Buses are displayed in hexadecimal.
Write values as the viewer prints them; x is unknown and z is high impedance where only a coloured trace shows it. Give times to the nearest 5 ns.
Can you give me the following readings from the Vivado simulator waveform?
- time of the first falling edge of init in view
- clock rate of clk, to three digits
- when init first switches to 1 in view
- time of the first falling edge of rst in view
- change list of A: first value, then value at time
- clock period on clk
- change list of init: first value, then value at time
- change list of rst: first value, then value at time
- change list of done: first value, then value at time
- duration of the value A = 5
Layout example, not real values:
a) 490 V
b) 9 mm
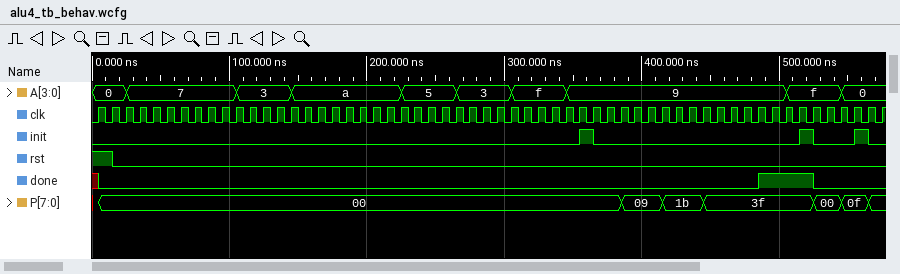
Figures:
a) 365 ns
b) 100 MHz
c) 355 ns
d) 15 ns
e) 0, 7 at 25 ns, 3 at 105 ns, a at 145 ns, 5 at 225 ns, 3 at 265 ns, f at 305 ns, 9 at 345 ns, f at 505 ns, 0 at 545 ns
f) 10 ns
g) 0, 1 at 355 ns, 0 at 365 ns, 1 at 515 ns, 0 at 525 ns, 1 at 555 ns, 0 at 565 ns
h) 1, 0 at 15 ns
i) x, 0 at 5 ns, 1 at 485 ns, 0 at 525 ns
j) 40 ns
